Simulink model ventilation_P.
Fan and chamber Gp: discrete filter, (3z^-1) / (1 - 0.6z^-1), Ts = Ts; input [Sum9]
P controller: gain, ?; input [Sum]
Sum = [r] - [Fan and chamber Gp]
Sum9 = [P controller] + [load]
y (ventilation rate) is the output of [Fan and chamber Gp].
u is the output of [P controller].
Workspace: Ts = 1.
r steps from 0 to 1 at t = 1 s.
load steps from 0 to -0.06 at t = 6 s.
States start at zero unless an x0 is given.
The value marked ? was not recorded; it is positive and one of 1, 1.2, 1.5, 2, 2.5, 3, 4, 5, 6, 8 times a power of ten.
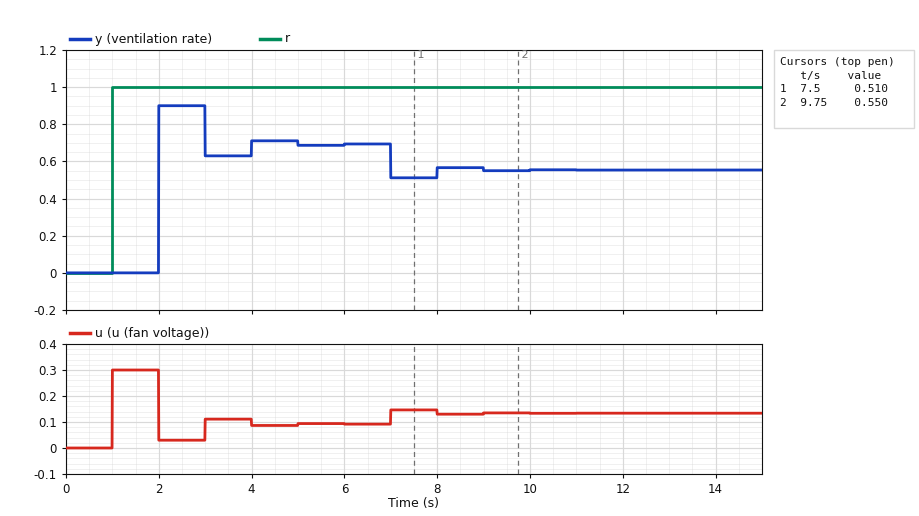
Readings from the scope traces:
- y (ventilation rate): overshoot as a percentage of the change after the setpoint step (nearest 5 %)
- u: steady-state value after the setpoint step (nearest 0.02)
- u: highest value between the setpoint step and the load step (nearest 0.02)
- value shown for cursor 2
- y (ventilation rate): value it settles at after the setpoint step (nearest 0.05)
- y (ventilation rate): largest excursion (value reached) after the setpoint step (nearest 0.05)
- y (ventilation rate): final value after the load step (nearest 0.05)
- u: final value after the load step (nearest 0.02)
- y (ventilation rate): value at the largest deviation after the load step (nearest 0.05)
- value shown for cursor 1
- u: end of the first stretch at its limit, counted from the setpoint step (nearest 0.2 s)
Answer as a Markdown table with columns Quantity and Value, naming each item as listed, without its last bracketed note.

| Quantity | Value |
|---|---|
| y (ventilation rate): overshoot as a percentage of the change after the setpoint step | 30 % |
| u: steady-state value after the setpoint step | 0.10 |
| u: highest value between the setpoint step and the load step | 0.30 |
| value shown for cursor 2 | 0.550 |
| y (ventilation rate): value it settles at after the setpoint step | 0.70 |
| y (ventilation rate): largest excursion (value reached) after the setpoint step | 0.90 |
| y (ventilation rate): final value after the load step | 0.55 |
| u: final value after the load step | 0.14 |
| y (ventilation rate): value at the largest deviation after the load step | 0.50 |
| value shown for cursor 1 | 0.510 |
| u: end of the first stretch at its limit, counted from the setpoint step | 1.0 s |
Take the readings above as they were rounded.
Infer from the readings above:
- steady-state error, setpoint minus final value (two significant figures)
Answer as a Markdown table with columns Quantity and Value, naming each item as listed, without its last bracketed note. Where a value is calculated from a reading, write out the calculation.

| Quantity | Value |
|---|---|
| steady-state error, setpoint minus final value | 1 - 0.7 = 0.30 |
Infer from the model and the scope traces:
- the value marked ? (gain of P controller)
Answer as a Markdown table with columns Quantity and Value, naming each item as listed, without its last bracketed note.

| Quantity | Value |
|---|---|
| the value marked ? | 0.3 |
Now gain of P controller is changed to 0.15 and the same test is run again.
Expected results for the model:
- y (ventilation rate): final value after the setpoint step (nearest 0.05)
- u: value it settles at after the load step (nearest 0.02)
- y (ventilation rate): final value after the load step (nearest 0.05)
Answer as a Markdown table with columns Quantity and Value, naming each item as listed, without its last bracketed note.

| Quantity | Value |
|---|---|
| y (ventilation rate): final value after the setpoint step | 0.55 |
| u: value it settles at after the load step | 0.10 |
| y (ventilation rate): final value after the load step | 0.30 |
